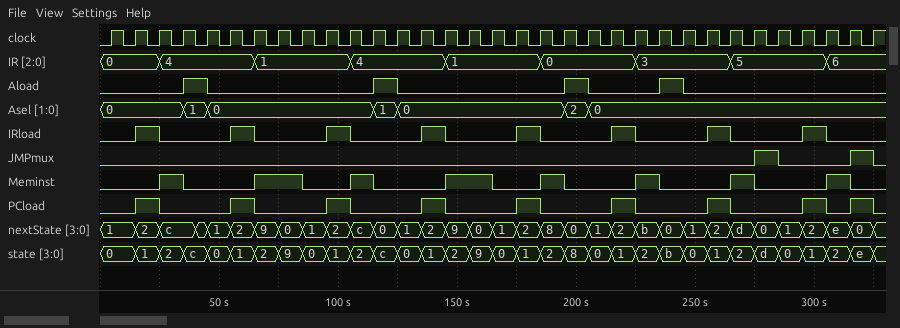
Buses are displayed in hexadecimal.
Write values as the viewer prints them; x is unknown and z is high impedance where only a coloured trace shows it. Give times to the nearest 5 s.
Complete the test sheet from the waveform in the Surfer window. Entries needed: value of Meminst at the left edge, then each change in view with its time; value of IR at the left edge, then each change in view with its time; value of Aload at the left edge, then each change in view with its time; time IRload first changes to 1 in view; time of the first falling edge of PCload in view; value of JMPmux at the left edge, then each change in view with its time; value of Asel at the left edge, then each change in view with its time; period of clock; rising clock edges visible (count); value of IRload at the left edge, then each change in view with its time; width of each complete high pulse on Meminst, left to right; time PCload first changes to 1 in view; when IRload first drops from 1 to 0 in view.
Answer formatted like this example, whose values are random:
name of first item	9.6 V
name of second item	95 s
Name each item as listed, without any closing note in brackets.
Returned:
value of Meminst at the left edge, then each change in view with its time	0, 1 at 25 s, 0 at 35 s, 1 at 65 s, 0 at 85 s, 1 at 105 s, 0 at 115 s, 1 at 145 s, 0 at 165 s, 1 at 185 s, 0 at 195 s, 1 at 225 s, 0 at 235 s, 1 at 265 s, 0 at 275 s, 1 at 305 s, 0 at 315 s
value of IR at the left edge, then each change in view with its time	0, 4 at 25 s, 1 at 65 s, 4 at 105 s, 1 at 145 s, 0 at 185 s, 3 at 225 s, 5 at 265 s, 6 at 305 s
value of Aload at the left edge, then each change in view with its time	0, 1 at 35 s, 0 at 45 s, 1 at 115 s, 0 at 125 s, 1 at 195 s, 0 at 205 s, 1 at 235 s, 0 at 245 s
time IRload first changes to 1 in view	15 s
time of the first falling edge of PCload in view	25 s
value of JMPmux at the left edge, then each change in view with its time	0, 1 at 275 s, 0 at 285 s, 1 at 315 s, 0 at 325 s
value of Asel at the left edge, then each change in view with its time	0, 1 at 35 s, 0 at 45 s, 1 at 115 s, 0 at 125 s, 2 at 195 s, 0 at 205 s
period of clock	10 s
rising clock edges visible	33
value of IRload at the left edge, then each change in view with its time	0, 1 at 15 s, 0 at 25 s, 1 at 55 s, 0 at 65 s, 1 at 95 s, 0 at 105 s, 1 at 135 s, 0 at 145 s, 1 at 175 s, 0 at 185 s, 1 at 215 s, 0 at 225 s, 1 at 255 s, 0 at 265 s, 1 at 295 s, 0 at 305 s
width of each complete high pulse on Meminst, left to right	10 s, 20 s, 10 s, 20 s, 10 s, 10 s, 10 s, 10 s
time PCload first changes to 1 in view	15 s
when IRload first drops from 1 to 0 in view	25 s
